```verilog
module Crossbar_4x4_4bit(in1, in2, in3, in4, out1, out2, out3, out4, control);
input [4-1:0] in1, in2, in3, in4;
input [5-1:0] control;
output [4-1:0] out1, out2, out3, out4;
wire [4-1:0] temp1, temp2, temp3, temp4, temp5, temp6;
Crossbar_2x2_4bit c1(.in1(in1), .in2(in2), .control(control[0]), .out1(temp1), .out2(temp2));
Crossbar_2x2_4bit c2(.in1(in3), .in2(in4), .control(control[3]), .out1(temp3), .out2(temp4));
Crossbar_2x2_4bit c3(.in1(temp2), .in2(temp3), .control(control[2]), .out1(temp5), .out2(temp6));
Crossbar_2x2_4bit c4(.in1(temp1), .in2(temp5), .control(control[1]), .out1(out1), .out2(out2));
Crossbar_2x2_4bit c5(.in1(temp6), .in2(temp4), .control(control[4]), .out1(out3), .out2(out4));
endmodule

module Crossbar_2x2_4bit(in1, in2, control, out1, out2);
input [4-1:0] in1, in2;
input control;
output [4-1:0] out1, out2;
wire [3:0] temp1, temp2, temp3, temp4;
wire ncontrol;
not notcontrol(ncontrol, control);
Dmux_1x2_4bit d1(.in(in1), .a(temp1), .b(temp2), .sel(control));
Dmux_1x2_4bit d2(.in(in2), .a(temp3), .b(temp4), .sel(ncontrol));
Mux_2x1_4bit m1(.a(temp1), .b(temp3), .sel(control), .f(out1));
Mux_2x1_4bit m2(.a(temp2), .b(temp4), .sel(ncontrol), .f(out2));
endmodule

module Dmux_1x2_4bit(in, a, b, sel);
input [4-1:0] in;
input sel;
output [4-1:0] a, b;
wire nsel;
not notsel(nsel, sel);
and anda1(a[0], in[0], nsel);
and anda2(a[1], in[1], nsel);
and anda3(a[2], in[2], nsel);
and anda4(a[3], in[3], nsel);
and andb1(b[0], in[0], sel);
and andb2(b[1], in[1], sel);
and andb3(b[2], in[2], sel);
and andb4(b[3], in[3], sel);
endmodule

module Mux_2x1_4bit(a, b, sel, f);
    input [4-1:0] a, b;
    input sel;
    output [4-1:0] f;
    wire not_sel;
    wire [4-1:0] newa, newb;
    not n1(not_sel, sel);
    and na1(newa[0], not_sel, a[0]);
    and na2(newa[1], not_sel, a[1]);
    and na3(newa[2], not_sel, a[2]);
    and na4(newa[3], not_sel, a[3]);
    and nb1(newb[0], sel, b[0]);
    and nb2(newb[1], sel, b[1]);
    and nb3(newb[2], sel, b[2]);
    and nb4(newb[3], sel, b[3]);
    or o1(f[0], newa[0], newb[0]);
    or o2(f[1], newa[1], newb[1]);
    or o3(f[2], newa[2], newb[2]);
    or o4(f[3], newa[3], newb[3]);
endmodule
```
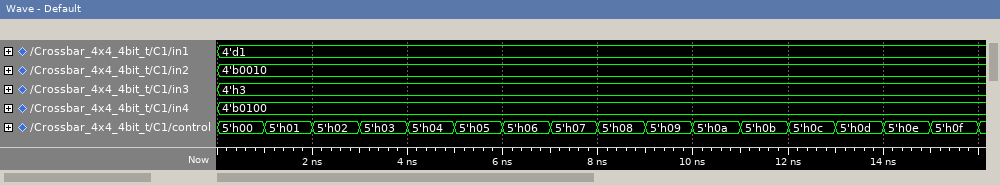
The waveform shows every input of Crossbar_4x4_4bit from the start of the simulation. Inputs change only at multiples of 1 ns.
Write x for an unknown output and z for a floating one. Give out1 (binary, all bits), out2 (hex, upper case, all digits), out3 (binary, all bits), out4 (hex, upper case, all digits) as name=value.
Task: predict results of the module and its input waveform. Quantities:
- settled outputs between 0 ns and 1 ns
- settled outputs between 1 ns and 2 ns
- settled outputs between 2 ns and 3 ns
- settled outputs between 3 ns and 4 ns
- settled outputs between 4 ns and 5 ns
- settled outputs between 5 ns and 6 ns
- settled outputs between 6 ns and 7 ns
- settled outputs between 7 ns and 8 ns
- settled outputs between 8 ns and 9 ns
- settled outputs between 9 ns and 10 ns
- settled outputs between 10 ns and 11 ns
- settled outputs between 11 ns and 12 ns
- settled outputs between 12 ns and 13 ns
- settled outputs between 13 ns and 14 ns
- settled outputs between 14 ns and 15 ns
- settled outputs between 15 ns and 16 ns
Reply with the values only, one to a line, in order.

out1=0001, out2=2, out3=0011, out4=4
out1=0010, out2=1, out3=0011, out4=4
out1=0010, out2=1, out3=0011, out4=4
out1=0001, out2=2, out3=0011, out4=4
out1=0001, out2=3, out3=0010, out4=4
out1=0010, out2=3, out3=0001, out4=4
out1=0011, out2=1, out3=0010, out4=4
out1=0011, out2=2, out3=0001, out4=4
out1=0001, out2=2, out3=0100, out4=3
out1=0010, out2=1, out3=0100, out4=3
out1=0010, out2=1, out3=0100, out4=3
out1=0001, out2=2, out3=0100, out4=3
out1=0001, out2=4, out3=0010, out4=3
out1=0010, out2=4, out3=0001, out4=3
out1=0100, out2=1, out3=0010, out4=3
out1=0100, out2=2, out3=0001, out4=3
